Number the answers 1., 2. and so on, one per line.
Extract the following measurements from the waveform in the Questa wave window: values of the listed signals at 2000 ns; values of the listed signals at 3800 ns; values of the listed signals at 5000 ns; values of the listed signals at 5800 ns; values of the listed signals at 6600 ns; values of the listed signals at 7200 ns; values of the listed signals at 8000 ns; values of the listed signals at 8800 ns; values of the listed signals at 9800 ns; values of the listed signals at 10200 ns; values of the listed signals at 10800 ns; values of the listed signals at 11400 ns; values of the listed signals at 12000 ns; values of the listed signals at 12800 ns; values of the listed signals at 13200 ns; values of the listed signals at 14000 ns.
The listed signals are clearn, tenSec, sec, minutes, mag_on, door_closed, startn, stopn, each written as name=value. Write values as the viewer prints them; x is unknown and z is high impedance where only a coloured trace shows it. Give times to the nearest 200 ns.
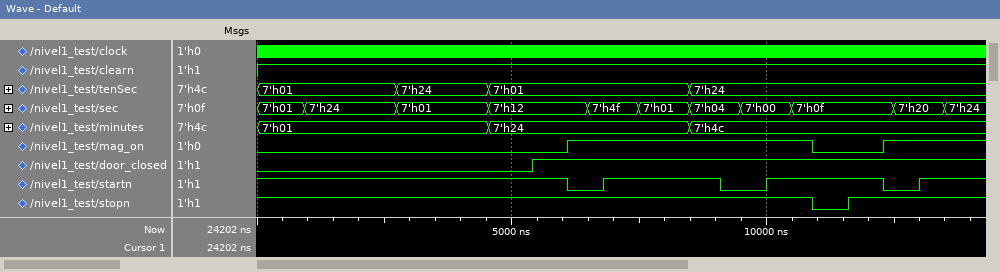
1. clearn=1, tenSec=7'h01, sec=7'h24, minutes=7'h01, mag_on=0, door_closed=0, startn=1, stopn=1
2. clearn=1, tenSec=7'h24, sec=7'h01, minutes=7'h01, mag_on=0, door_closed=0, startn=1, stopn=1
3. clearn=1, tenSec=7'h01, sec=7'h12, minutes=7'h24, mag_on=0, door_closed=0, startn=1, stopn=1
4. clearn=1, tenSec=7'h01, sec=7'h12, minutes=7'h24, mag_on=0, door_closed=1, startn=1, stopn=1
5. clearn=1, tenSec=7'h01, sec=7'h4f, minutes=7'h24, mag_on=1, door_closed=1, startn=0, stopn=1
6. clearn=1, tenSec=7'h01, sec=7'h4f, minutes=7'h24, mag_on=1, door_closed=1, startn=1, stopn=1
7. clearn=1, tenSec=7'h01, sec=7'h01, minutes=7'h24, mag_on=1, door_closed=1, startn=1, stopn=1
8. clearn=1, tenSec=7'h24, sec=7'h04, minutes=7'h4c, mag_on=1, door_closed=1, startn=1, stopn=1
9. clearn=1, tenSec=7'h24, sec=7'h00, minutes=7'h4c, mag_on=1, door_closed=1, startn=0, stopn=1
10. clearn=1, tenSec=7'h24, sec=7'h00, minutes=7'h4c, mag_on=1, door_closed=1, startn=1, stopn=1
11. clearn=1, tenSec=7'h24, sec=7'h0f, minutes=7'h4c, mag_on=1, door_closed=1, startn=1, stopn=1
12. clearn=1, tenSec=7'h24, sec=7'h0f, minutes=7'h4c, mag_on=0, door_closed=1, startn=1, stopn=0
13. clearn=1, tenSec=7'h24, sec=7'h0f, minutes=7'h4c, mag_on=0, door_closed=1, startn=1, stopn=1
14. clearn=1, tenSec=7'h24, sec=7'h20, minutes=7'h4c, mag_on=1, door_closed=1, startn=0, stopn=1
15. clearn=1, tenSec=7'h24, sec=7'h20, minutes=7'h4c, mag_on=1, door_closed=1, startn=1, stopn=1
16. clearn=1, tenSec=7'h24, sec=7'h24, minutes=7'h4c, mag_on=1, door_closed=1, startn=1, stopn=1
